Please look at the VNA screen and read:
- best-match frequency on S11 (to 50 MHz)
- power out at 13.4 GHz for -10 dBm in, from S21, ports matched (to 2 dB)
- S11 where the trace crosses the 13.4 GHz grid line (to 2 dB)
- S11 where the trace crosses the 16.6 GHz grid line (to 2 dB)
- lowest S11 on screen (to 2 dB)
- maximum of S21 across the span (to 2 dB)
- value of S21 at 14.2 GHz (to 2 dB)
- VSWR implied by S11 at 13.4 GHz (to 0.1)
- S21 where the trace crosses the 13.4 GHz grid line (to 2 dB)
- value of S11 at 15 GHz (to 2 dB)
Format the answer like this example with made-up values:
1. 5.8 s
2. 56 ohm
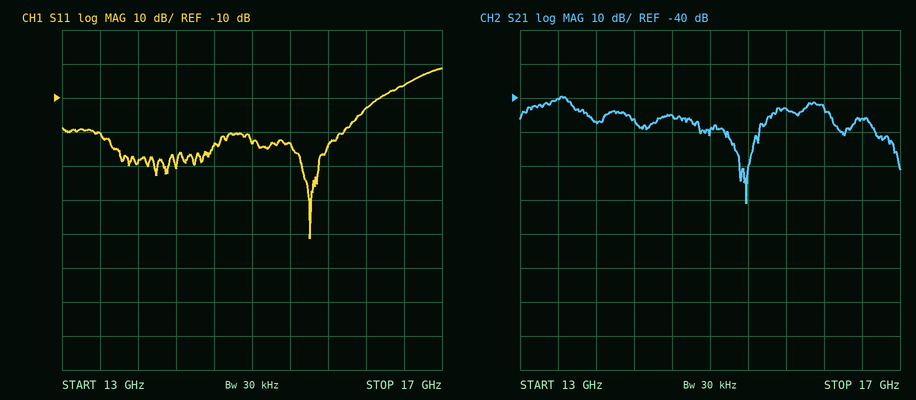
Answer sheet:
1. 15.60 GHz
2. -50 dBm
3. -20 dB
4. -6 dB
5. -52 dB
6. -40 dB
7. -46 dB
8. 1.2
9. -40 dB
10. -24 dB
